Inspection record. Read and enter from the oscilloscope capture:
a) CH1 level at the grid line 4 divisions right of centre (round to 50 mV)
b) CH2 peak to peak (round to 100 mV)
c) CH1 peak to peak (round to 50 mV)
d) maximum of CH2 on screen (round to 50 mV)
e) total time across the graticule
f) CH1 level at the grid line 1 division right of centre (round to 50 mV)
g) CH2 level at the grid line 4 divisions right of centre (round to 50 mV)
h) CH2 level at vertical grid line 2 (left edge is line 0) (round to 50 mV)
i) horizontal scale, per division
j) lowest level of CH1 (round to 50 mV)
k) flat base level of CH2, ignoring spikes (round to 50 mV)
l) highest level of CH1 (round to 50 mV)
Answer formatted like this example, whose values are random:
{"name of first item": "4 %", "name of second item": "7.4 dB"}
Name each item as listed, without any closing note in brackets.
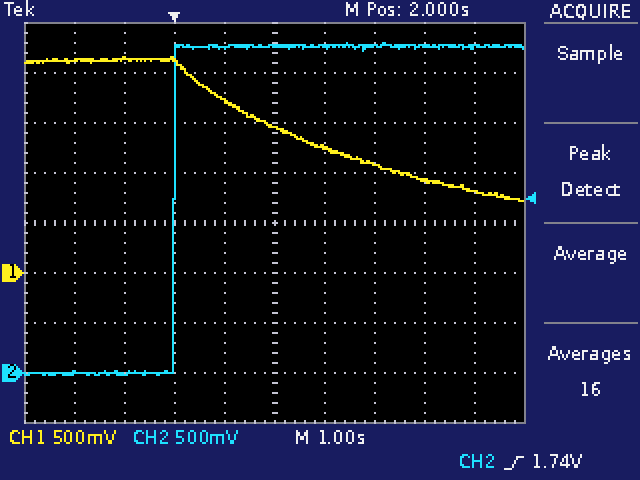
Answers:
{"CH1 level at the grid line 4 divisions right of centre": "800 mV", "CH2 peak to peak": "3.30 V", "CH1 peak to peak": "1.45 V", "maximum of CH2 on screen": "3.30 V", "total time across the graticule": "10 s", "CH1 level at the grid line 1 division right of centre": "1.25 V", "CH2 level at the grid line 4 divisions right of centre": "3.25 V", "CH2 level at vertical grid line 2 (left edge is line 0)": "0 mV", "horizontal scale, per division": "1 s", "lowest level of CH1": "700 mV", "flat base level of CH2, ignoring spikes": "0 mV", "highest level of CH1": "2.15 V"}
